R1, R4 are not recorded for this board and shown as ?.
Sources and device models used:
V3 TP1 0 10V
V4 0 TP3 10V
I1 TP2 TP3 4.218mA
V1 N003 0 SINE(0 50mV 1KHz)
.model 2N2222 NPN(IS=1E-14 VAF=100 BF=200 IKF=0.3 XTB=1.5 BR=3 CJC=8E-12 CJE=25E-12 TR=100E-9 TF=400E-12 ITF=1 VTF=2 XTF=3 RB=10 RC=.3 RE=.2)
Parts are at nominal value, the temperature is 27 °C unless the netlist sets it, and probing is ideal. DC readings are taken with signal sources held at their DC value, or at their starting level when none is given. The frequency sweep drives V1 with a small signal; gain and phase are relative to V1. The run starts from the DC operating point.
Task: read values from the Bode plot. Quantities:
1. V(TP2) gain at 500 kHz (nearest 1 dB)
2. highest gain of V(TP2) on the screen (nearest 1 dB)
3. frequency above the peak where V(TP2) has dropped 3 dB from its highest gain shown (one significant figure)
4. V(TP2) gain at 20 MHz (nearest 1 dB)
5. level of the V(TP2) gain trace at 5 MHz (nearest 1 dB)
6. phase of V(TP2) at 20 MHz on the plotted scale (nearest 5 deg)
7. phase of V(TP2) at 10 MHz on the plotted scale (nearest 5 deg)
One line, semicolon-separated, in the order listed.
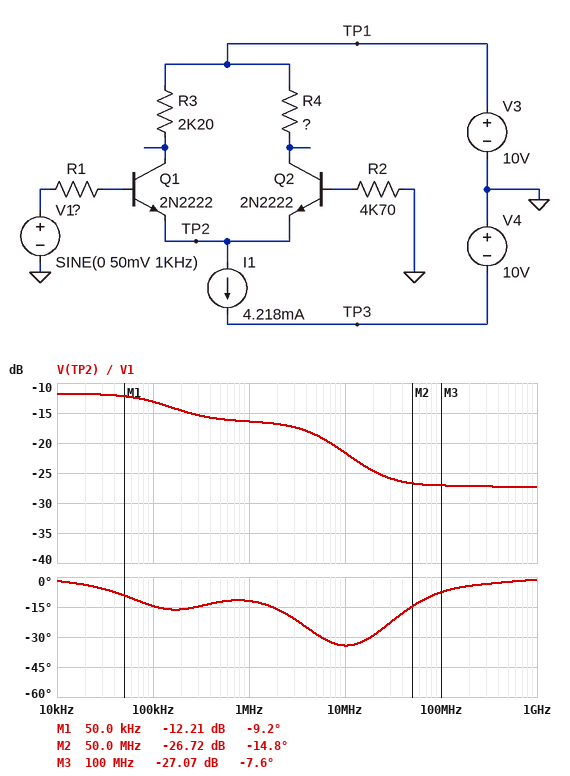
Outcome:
-16 dB; -12 dB; 200 kHz; -25 dB; -19 dB; -30 deg; -35 deg
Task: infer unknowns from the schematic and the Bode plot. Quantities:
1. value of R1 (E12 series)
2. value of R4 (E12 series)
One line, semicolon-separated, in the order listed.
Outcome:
15 kΩ; 1.2 kΩ
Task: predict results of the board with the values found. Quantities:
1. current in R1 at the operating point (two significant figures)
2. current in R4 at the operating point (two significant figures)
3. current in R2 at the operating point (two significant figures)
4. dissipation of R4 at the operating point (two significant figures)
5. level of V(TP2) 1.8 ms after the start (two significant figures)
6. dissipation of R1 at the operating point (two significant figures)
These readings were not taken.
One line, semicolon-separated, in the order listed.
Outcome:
5.9 µA; 2.9 mA; 14 µA; 10 mW; -760 mV; 520 nW
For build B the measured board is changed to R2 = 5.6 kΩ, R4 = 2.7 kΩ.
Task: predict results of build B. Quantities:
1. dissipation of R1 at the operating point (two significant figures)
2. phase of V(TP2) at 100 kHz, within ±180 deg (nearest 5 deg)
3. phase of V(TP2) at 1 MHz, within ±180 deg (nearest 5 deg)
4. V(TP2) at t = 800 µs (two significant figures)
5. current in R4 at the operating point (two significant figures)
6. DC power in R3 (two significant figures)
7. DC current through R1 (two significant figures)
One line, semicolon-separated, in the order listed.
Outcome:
630 nW; 5 deg; -15 deg; -770 mV; 2.8 mA; 4.2 mW; 6.5 µA
